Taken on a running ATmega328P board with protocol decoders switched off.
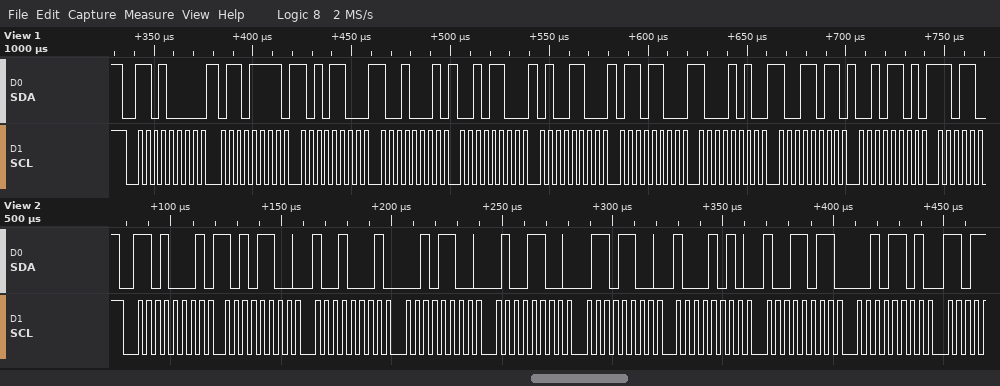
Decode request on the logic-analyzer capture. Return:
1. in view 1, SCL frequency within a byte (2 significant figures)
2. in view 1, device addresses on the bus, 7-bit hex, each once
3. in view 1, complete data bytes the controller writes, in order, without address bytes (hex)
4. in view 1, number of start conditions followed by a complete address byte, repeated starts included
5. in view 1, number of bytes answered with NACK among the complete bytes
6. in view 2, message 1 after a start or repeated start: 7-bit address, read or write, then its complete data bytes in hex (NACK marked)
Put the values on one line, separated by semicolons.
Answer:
250 kHz; 0x68; 6F AC 91 2C 4C 6C 8A 9B 2D; 1; 0; 0x68 read: AC 91 2C 4C 6C 8A 9B 2D
